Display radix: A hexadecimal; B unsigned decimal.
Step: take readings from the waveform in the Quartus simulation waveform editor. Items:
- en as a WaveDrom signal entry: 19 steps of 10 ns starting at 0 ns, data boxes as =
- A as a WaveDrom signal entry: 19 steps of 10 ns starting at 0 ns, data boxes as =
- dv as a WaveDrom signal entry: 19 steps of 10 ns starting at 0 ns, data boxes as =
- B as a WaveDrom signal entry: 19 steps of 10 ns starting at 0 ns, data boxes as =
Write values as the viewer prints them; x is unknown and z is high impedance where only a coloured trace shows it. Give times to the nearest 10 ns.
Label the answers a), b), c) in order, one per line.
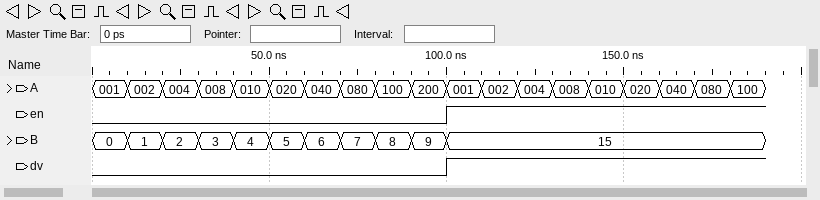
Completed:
a) {name: 'en', wave: '0.........1........'}
b) {name: 'A', wave: '===================', data: '001 002 004 008 010 020 040 080 100 200 001 002 004 008 010 020 040 080 100'}
c) {name: 'dv', wave: '0.........1........'}
d) {name: 'B', wave: '===========........', data: '0 1 2 3 4 5 6 7 8 9 15'}
